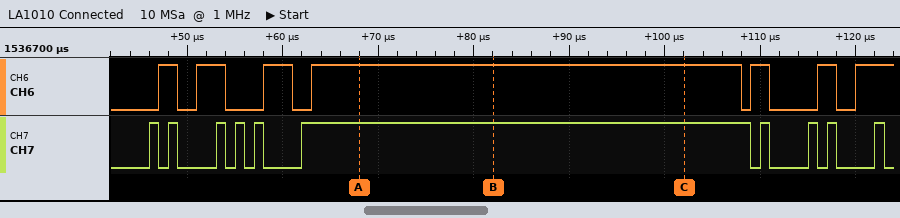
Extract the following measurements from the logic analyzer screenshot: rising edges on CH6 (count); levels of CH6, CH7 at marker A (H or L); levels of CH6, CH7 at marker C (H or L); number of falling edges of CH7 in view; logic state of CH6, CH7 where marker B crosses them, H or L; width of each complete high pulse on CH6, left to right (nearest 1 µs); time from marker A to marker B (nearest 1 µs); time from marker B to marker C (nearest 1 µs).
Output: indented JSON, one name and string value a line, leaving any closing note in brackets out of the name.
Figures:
{
  "rising edges on CH6": "7",
  "levels of CH6, CH7 at marker A": "CH6=H, CH7=H",
  "levels of CH6, CH7 at marker C": "CH6=H, CH7=H",
  "number of falling edges of CH7 in view": "10",
  "logic state of CH6, CH7 where marker B crosses them, H or L": "CH6=H, CH7=H",
  "width of each complete high pulse on CH6, left to right": "2 µs, 3 µs, 3 µs, 45 µs, 2 µs, 2 µs",
  "time from marker A to marker B": "14 µs",
  "time from marker B to marker C": "20 µs"
}
